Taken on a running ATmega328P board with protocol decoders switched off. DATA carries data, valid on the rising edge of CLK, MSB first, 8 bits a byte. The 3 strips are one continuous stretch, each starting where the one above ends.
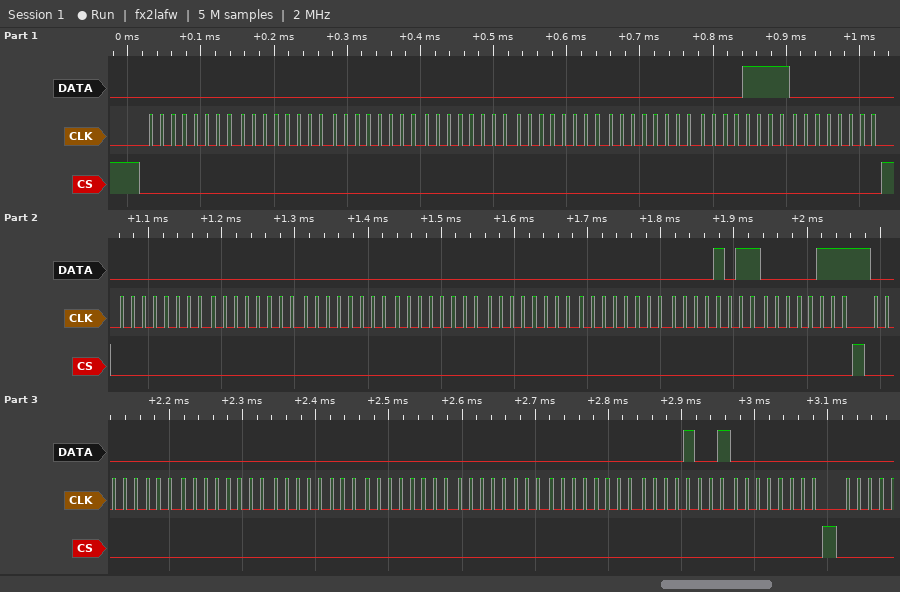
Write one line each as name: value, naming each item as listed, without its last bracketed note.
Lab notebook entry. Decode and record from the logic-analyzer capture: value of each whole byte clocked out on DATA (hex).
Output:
value of each whole byte clocked out on DATA: 00 00 00 00 00 00 0F 00 00 00 00 00 00 00 0B 07 00 00 00 00 00 00 09 00
